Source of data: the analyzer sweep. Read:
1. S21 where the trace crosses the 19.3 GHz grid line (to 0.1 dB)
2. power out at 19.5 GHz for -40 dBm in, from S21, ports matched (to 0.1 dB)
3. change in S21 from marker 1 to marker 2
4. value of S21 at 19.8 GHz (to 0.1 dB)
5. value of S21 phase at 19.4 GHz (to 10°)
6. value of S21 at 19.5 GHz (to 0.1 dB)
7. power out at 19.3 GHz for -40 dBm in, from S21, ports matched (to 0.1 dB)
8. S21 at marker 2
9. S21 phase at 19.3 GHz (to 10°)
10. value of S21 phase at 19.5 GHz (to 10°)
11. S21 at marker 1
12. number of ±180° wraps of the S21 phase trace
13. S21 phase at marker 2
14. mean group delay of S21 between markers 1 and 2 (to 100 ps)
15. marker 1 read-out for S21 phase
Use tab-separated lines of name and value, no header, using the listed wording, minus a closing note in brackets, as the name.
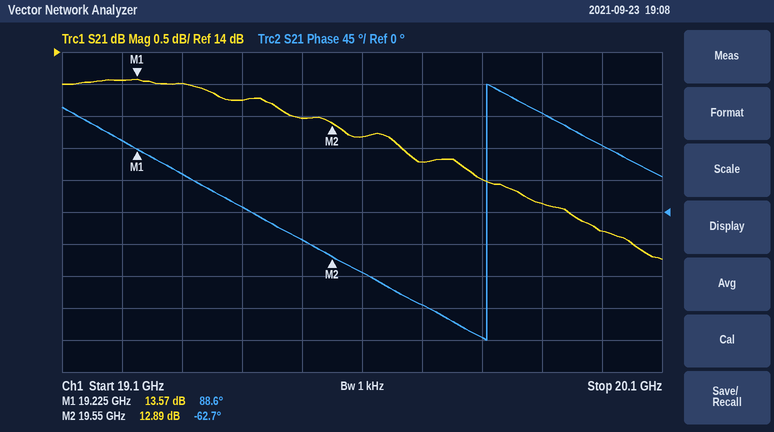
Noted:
S21 where the trace crosses the 19.3 GHz grid line	13.5 dB
power out at 19.5 GHz for -40 dBm in, from S21, ports matched	-27.0 dBm
change in S21 from marker 1 to marker 2	-0.68 dB
value of S21 at 19.8 GHz	12.0 dB
value of S21 phase at 19.4 GHz	10°
value of S21 at 19.5 GHz	13.0 dB
power out at 19.3 GHz for -40 dBm in, from S21, ports matched	-26.5 dBm
S21 at marker 2	12.89 dB
S21 phase at 19.3 GHz	50°
value of S21 phase at 19.5 GHz	-40°
S21 at marker 1	13.57 dB
number of ±180° wraps of the S21 phase trace	1
S21 phase at marker 2	-62.7°
mean group delay of S21 between markers 1 and 2	1.3 ns
marker 1 read-out for S21 phase	88.6°
